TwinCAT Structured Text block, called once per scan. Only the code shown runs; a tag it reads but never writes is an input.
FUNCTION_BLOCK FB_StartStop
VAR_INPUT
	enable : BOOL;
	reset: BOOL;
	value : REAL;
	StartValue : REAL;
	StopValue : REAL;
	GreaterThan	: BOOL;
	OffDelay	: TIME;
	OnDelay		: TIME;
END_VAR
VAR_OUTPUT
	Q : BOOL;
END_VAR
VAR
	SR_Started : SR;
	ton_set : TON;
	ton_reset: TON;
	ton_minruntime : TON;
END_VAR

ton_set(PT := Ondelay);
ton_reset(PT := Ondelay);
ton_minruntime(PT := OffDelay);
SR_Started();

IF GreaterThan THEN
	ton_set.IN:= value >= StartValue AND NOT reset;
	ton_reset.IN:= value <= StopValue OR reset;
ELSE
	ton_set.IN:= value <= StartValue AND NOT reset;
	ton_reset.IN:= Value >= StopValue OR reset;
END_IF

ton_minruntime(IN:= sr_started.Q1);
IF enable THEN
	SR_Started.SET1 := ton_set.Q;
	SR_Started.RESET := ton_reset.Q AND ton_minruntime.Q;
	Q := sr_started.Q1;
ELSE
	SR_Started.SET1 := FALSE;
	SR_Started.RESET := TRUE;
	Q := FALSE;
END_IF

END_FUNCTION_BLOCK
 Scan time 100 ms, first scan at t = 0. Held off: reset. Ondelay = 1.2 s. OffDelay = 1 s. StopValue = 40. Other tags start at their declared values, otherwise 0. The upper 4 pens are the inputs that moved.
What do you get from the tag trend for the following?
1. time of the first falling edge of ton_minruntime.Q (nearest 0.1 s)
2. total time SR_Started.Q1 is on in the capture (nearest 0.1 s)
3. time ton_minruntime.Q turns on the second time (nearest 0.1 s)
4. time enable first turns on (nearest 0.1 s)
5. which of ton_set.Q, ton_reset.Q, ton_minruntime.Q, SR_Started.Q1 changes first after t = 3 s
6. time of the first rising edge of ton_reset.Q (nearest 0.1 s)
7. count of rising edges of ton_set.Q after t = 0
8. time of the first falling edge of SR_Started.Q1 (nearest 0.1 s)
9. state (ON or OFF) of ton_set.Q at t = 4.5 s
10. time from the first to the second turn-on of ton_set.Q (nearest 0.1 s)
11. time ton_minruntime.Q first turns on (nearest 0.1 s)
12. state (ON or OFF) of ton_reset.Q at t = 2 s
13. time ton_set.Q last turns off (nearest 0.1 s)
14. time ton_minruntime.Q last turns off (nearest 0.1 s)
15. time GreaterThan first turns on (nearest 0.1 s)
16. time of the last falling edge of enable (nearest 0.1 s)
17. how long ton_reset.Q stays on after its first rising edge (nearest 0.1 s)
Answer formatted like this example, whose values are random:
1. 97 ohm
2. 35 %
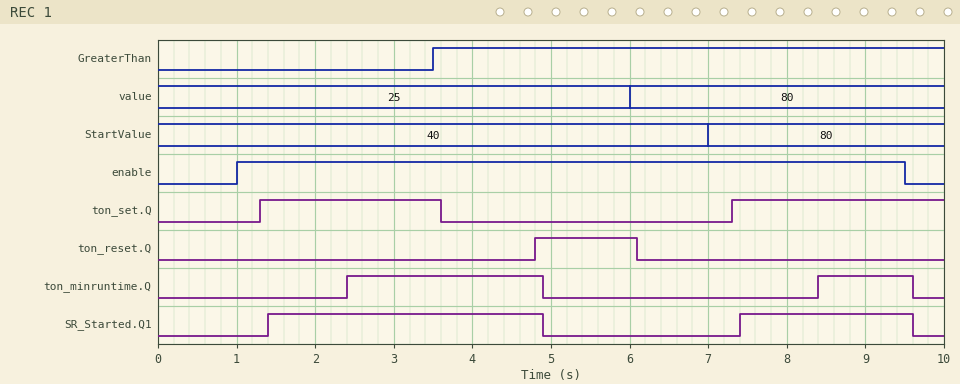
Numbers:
1. 4.9 s
2. 5.7 s
3. 8.4 s
4. 1.0 s
5. ton_set.Q
6. 4.8 s
7. 2
8. 4.9 s
9. OFF
10. 6.0 s
11. 2.4 s
12. OFF
13. 3.6 s
14. 9.6 s
15. 3.5 s
16. 9.5 s
17. 1.3 s
